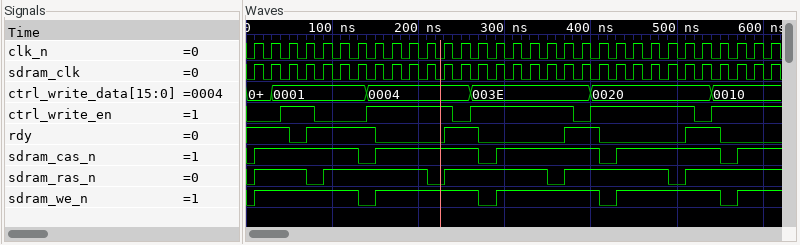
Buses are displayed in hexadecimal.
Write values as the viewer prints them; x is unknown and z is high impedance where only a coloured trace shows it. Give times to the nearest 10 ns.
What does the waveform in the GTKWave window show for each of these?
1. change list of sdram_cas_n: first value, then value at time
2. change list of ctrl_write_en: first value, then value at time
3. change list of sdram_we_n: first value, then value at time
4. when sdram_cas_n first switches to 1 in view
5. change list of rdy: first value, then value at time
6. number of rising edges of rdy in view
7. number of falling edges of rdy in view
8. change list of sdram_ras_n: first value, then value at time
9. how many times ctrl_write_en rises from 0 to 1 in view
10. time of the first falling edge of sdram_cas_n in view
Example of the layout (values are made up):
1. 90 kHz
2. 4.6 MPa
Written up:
1. 0, 1 at 10 ns, 0 at 130 ns, 1 at 150 ns, 0 at 270 ns, 1 at 290 ns, 0 at 410 ns, 1 at 430 ns, 0 at 550 ns, 1 at 570 ns
2. 0, 1 at 40 ns, 0 at 80 ns, 1 at 140 ns, 0 at 240 ns, 1 at 260 ns, 0 at 380 ns, 1 at 400 ns, 0 at 520 ns, 1 at 540 ns
3. 0, 1 at 10 ns, 0 at 130 ns, 1 at 150 ns, 0 at 270 ns, 1 at 290 ns, 0 at 410 ns, 1 at 430 ns, 0 at 550 ns, 1 at 570 ns
4. 10 ns
5. 1, 0 at 50 ns, 1 at 70 ns, 0 at 150 ns, 1 at 230 ns, 0 at 270 ns, 1 at 370 ns, 0 at 410 ns, 1 at 510 ns, 0 at 550 ns
6. 4
7. 5
8. 0, 1 at 10 ns, 0 at 70 ns, 1 at 90 ns, 0 at 210 ns, 1 at 230 ns, 0 at 350 ns, 1 at 370 ns, 0 at 490 ns, 1 at 510 ns
9. 5
10. 130 ns
